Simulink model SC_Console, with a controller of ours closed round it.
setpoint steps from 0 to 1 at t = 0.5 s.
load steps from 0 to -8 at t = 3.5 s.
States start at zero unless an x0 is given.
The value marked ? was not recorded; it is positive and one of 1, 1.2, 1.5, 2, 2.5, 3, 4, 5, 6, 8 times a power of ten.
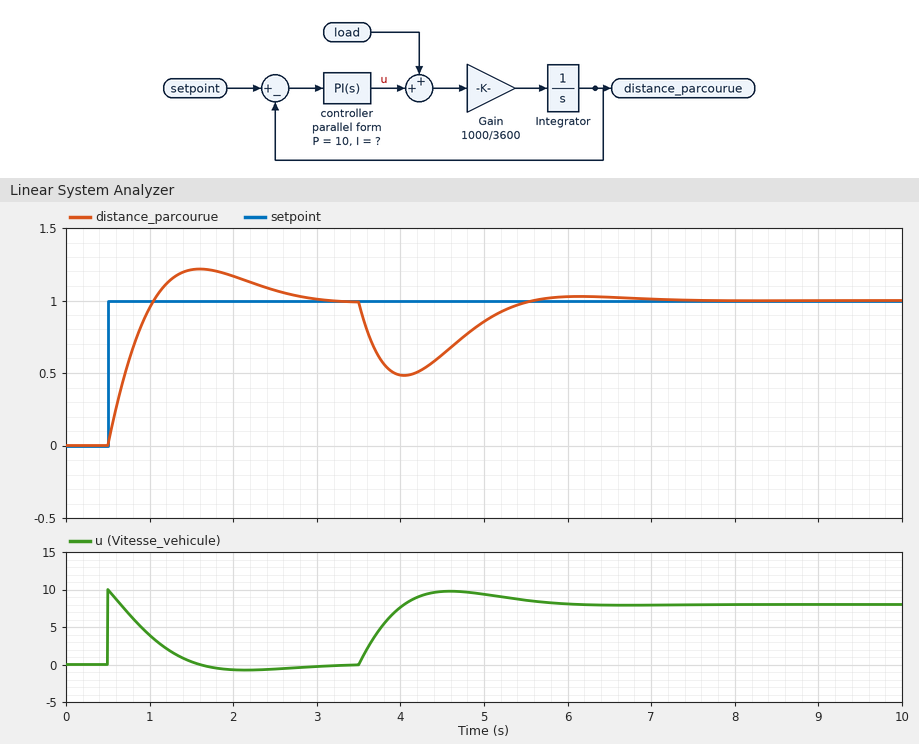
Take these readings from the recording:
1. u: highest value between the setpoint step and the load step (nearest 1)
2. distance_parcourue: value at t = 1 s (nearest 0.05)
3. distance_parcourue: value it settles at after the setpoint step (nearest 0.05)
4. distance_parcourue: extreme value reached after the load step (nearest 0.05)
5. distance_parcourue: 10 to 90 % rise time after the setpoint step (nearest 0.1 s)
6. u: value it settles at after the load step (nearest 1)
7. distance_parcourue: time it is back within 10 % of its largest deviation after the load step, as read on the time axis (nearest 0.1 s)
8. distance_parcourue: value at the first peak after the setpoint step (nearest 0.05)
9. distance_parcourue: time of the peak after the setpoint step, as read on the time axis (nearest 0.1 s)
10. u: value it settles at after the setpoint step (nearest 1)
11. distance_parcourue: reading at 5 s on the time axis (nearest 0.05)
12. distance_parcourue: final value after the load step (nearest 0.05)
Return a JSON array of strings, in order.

["10", "0.95", "1.00", "0.50", "0.4 s", "8", "5.3 s", "1.20", "1.6 s", "0", "0.85", "1.00"]
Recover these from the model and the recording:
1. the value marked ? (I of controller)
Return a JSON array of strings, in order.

["15"]
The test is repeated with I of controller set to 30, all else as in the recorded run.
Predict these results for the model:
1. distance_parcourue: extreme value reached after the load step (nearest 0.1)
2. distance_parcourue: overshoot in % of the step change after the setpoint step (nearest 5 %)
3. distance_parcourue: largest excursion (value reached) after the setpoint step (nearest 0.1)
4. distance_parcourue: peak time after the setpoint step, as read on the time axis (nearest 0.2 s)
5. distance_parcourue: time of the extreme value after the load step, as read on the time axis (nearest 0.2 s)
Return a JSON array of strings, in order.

["0.6", "30 %", "1.3", "1.4 s", "4.0 s"]
